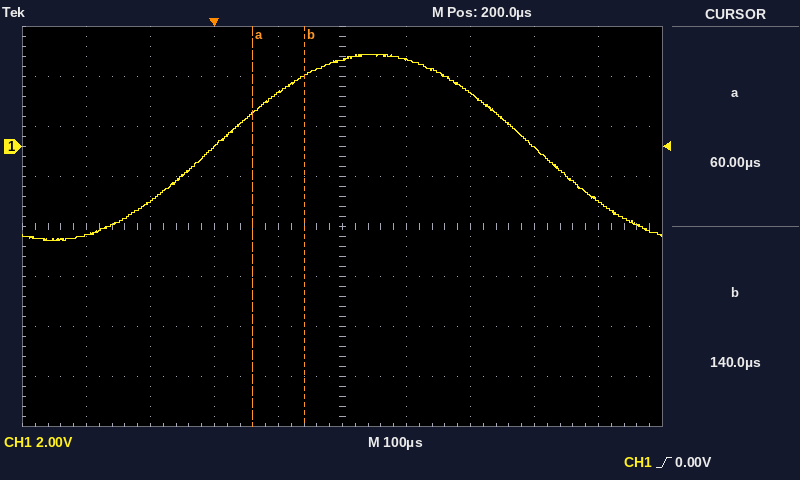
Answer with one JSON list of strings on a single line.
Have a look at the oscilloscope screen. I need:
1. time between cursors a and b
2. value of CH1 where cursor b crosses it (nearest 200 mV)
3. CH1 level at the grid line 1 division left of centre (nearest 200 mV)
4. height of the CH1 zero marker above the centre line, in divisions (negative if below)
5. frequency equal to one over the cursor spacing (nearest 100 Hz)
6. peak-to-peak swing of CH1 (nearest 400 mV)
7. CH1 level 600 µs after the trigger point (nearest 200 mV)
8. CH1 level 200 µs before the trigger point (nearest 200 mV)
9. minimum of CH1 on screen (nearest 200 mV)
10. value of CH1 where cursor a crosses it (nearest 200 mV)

["80 µs", "2.8 V", "2.2 V", "+1.6 div", "12.5 kHz", "7.6 V", "-2.2 V", "-3.6 V", "-3.8 V", "1.4 V"]
